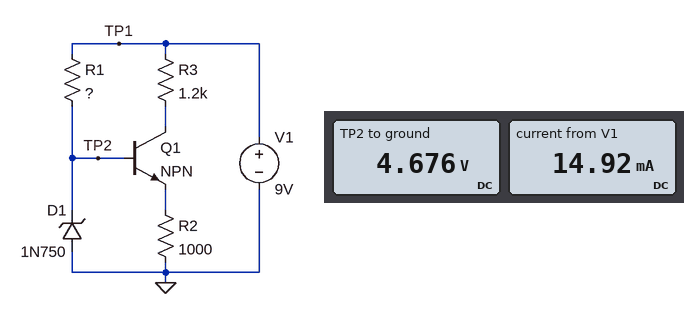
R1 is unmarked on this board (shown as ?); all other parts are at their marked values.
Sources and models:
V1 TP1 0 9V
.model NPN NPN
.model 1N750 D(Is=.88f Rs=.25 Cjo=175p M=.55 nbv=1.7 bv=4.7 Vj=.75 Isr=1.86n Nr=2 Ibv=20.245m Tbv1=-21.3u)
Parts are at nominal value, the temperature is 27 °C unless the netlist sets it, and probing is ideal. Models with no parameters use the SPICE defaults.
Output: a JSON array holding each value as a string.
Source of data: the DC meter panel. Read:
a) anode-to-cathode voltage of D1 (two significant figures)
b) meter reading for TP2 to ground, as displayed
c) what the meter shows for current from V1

["-4.7 V", "4.676 V", "14.92 mA"]
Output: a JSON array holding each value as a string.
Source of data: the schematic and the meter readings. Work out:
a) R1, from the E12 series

["390 Ω"]
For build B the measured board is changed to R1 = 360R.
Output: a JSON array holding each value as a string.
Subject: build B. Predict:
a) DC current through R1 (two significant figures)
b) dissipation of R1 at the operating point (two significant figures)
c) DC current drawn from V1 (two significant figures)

["12 mA", "52 mW", "16 mA"]
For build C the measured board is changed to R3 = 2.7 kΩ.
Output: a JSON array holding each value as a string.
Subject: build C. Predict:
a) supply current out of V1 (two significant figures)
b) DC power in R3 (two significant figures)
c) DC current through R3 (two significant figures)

["13 mA", "9.7 mW", "1.9 mA"]
